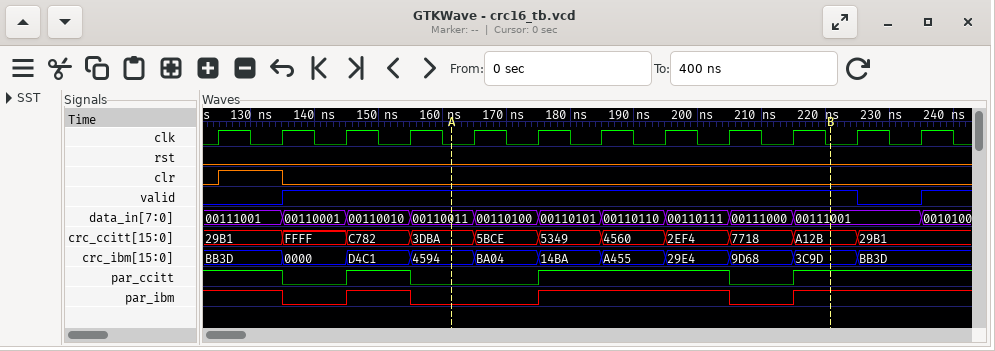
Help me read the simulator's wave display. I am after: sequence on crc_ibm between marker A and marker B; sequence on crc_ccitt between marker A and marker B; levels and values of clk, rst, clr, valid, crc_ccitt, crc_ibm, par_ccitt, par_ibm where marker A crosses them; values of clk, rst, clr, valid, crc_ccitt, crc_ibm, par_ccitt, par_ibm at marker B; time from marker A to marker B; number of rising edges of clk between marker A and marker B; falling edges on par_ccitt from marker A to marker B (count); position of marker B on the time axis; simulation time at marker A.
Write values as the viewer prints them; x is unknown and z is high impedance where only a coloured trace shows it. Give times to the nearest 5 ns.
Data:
4594, BA04, 14BA, A455, 29E4, 9D68, 3C9D
3DBA, 5BCE, 5349, 4560, 2EF4, 7718, A12B
clk=0, rst=0, clr=0, valid=1, crc_ccitt=3DBA, crc_ibm=4594, par_ccitt=0, par_ibm=0
clk=0, rst=0, clr=0, valid=1, crc_ccitt=A12B, crc_ibm=3C9D, par_ccitt=1, par_ibm=1
60 ns
6
1
220 ns
160 ns
